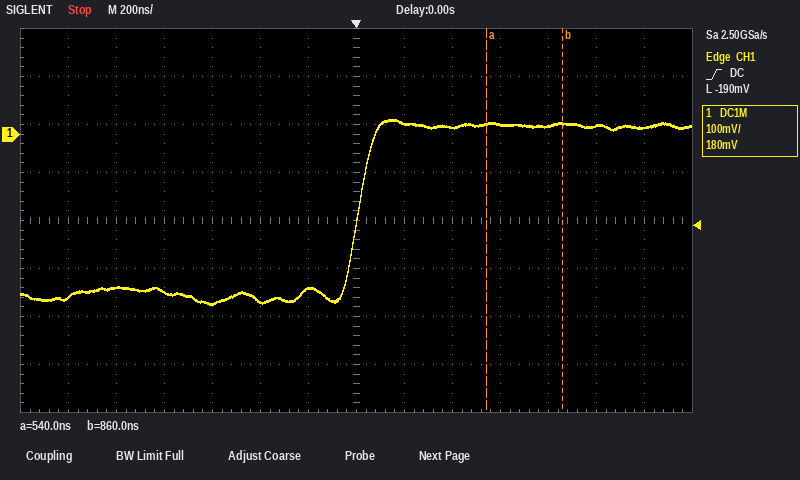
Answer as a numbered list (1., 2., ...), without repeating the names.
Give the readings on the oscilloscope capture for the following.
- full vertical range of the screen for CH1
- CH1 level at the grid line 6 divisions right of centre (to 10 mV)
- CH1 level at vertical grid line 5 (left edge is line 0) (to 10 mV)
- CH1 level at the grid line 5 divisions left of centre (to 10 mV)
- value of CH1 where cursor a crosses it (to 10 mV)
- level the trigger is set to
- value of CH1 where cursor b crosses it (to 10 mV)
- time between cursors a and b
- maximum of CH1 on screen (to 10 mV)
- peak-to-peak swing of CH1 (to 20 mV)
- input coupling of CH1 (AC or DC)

1. 800 mV
2. 10 mV
3. -350 mV
4. -320 mV
5. 20 mV
6. -190 mV
7. 20 mV
8. 320 ns
9. 30 mV
10. 380 mV
11. DC
